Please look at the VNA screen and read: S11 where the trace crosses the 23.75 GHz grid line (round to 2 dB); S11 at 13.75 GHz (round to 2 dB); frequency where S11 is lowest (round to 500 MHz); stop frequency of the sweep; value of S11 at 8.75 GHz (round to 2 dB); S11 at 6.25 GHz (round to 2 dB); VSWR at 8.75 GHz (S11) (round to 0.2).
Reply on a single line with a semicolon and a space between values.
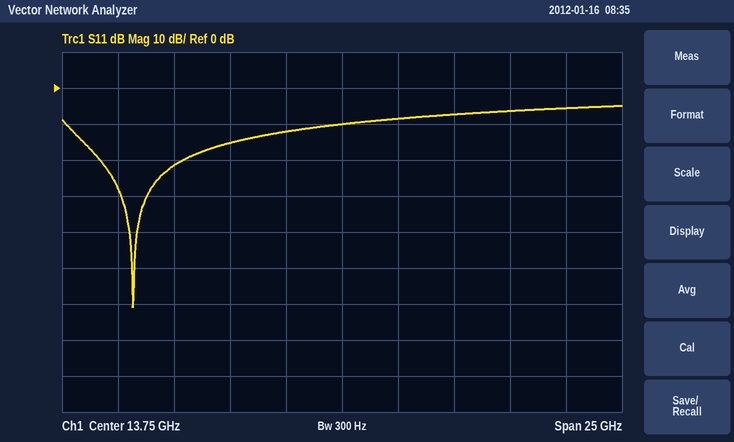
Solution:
-6 dB; -10 dB; 4.5 GHz; 26.25 GHz; -16 dB; -22 dB; 1.4
